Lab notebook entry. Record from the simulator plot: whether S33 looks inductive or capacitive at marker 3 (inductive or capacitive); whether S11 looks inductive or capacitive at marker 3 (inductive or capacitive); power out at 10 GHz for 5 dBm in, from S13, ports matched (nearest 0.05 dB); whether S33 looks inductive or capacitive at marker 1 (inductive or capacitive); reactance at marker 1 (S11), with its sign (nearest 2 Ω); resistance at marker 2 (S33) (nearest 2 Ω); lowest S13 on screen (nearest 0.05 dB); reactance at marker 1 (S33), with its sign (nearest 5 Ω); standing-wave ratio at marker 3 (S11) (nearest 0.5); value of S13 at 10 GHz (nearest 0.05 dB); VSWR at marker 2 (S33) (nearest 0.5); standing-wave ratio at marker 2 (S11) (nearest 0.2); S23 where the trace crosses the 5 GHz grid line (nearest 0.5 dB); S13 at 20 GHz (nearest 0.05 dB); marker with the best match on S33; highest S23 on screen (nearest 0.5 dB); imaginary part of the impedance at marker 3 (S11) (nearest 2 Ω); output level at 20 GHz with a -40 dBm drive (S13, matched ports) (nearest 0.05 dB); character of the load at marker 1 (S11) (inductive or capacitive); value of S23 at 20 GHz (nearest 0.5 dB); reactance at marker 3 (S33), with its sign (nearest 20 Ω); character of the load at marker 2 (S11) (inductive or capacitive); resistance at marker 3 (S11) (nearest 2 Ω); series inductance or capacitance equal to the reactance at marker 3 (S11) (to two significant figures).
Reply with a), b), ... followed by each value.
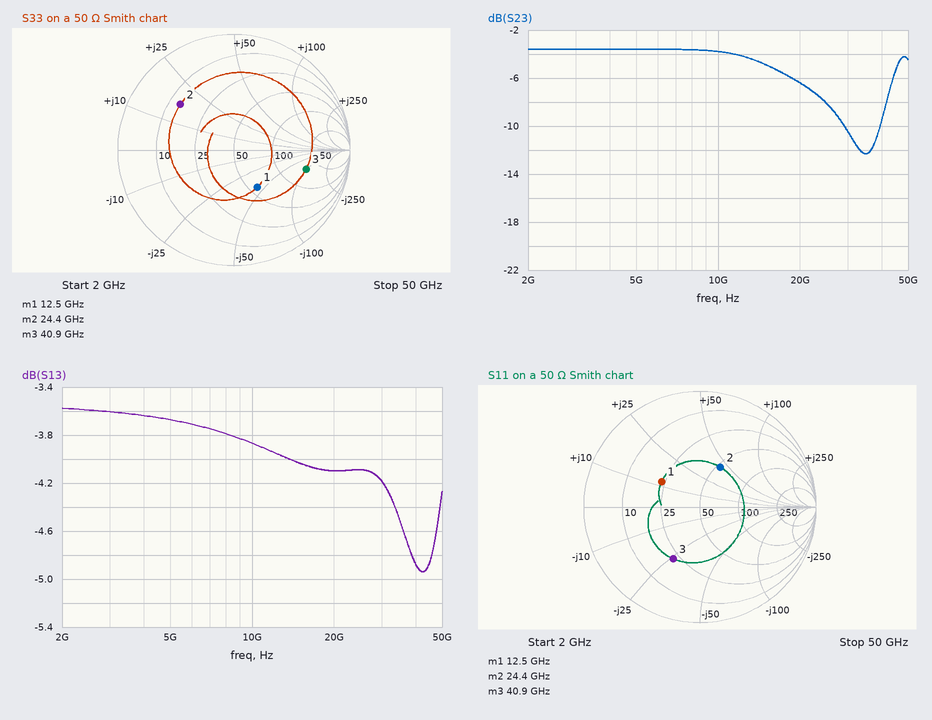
a) capacitive
b) capacitive
c) 1.15 dBm
d) capacitive
e) +12 Ω
f) 14 Ω
g) -4.95 dB
h) -45 Ω
i) 3.0
j) -3.85 dB
k) 4.0
l) 2.2
m) -3.5 dB
n) -4.10 dB
o) marker 1
p) -3.5 dB
q) -26 Ω
r) -44.10 dBm
s) inductive
t) -6.5 dB
u) -100 Ω
v) inductive
w) 22 Ω
x) 150 fF
